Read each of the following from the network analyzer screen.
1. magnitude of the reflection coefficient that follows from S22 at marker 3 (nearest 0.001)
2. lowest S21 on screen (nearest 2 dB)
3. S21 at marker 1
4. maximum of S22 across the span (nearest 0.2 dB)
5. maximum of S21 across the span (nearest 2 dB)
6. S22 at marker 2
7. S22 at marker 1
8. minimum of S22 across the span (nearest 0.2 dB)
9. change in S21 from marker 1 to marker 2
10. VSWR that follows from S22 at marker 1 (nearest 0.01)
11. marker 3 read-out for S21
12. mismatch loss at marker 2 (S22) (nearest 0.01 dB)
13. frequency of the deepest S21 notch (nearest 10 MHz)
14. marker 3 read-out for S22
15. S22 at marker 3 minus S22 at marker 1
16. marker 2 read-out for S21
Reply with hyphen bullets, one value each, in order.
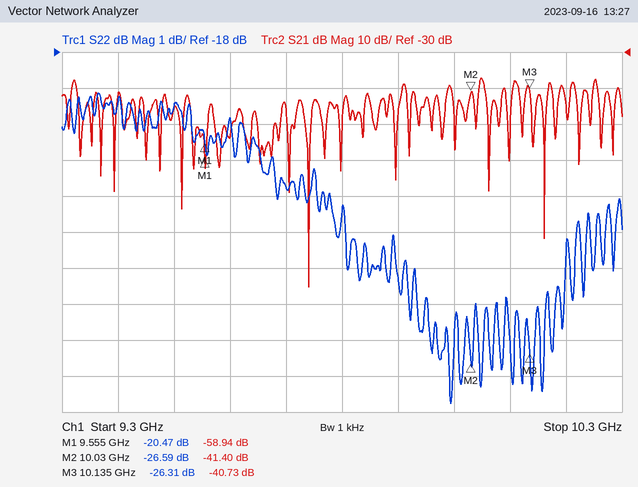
- 0.048
- -96 dB
- -58.94 dB
- -19.2 dB
- -38 dB
- -26.59 dB
- -20.47 dB
- -27.8 dB
- 17.54 dB
- 1.21
- -40.73 dB
- 0.01 dB
- 9.74 GHz
- -26.31 dB
- -5.84 dB
- -41.40 dB
